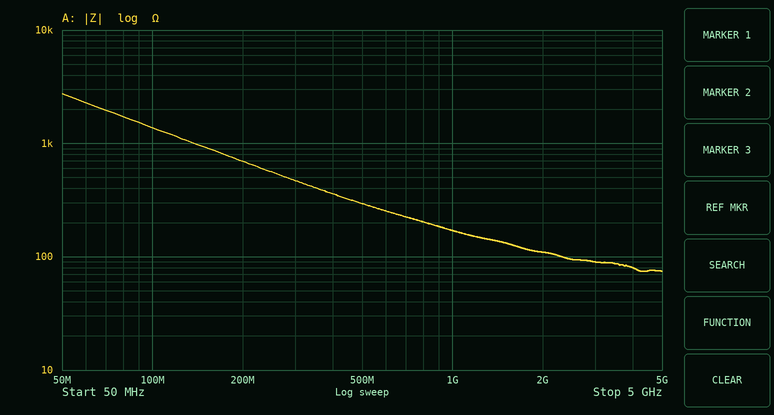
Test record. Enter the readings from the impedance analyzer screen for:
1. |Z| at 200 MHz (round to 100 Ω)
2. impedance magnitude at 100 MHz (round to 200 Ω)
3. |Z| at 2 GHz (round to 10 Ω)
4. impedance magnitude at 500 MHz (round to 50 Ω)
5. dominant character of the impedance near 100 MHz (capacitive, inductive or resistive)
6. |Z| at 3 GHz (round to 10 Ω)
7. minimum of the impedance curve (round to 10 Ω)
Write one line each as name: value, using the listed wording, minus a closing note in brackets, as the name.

|Z| at 200 MHz: 700 Ω
impedance magnitude at 100 MHz: 1.4 kΩ
|Z| at 2 GHz: 110 Ω
impedance magnitude at 500 MHz: 300 Ω
dominant character of the impedance near 100 MHz: capacitive
|Z| at 3 GHz: 90 Ω
minimum of the impedance curve: 70 Ω
